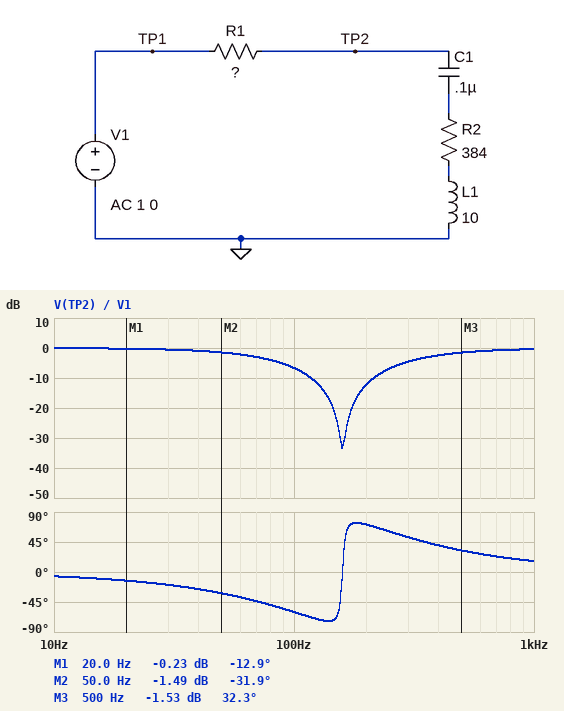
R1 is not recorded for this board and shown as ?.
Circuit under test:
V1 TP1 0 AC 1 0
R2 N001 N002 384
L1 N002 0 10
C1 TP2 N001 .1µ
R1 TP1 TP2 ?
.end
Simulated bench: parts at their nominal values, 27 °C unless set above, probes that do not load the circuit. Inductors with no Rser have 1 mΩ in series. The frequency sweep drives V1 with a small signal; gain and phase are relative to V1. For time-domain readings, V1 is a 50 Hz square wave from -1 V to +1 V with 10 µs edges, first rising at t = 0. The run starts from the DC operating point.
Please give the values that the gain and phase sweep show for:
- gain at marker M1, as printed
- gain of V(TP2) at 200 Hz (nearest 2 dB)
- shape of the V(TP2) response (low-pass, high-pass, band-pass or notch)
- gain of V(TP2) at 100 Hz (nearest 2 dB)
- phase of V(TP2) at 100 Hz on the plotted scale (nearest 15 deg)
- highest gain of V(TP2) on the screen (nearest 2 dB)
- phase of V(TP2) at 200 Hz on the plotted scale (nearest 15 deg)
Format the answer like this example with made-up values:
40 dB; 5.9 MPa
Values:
-0.23 dB; -12 dB; notch; -6 dB; -60 deg; 0 dB; 75 deg
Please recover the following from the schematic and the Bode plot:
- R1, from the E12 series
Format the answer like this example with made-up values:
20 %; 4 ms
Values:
18 kΩ
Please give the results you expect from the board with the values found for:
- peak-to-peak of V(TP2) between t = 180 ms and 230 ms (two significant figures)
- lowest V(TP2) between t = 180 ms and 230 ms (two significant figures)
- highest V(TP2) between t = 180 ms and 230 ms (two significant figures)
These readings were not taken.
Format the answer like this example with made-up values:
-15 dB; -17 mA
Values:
2.0 V; -1.0 V; 1.0 V
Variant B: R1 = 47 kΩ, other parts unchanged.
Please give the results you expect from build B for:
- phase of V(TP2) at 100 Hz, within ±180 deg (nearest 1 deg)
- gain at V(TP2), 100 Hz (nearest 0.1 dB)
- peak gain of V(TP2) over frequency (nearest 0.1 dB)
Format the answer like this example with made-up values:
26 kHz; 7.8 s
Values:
-76 deg; -14.0 dB; 0 dB
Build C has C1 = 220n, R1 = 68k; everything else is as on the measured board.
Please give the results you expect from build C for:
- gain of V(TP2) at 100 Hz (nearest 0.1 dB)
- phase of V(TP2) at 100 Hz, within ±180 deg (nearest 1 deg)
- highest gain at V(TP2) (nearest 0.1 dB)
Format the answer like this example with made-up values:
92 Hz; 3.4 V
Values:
-36.5 dB; -67 deg; 0 dB
